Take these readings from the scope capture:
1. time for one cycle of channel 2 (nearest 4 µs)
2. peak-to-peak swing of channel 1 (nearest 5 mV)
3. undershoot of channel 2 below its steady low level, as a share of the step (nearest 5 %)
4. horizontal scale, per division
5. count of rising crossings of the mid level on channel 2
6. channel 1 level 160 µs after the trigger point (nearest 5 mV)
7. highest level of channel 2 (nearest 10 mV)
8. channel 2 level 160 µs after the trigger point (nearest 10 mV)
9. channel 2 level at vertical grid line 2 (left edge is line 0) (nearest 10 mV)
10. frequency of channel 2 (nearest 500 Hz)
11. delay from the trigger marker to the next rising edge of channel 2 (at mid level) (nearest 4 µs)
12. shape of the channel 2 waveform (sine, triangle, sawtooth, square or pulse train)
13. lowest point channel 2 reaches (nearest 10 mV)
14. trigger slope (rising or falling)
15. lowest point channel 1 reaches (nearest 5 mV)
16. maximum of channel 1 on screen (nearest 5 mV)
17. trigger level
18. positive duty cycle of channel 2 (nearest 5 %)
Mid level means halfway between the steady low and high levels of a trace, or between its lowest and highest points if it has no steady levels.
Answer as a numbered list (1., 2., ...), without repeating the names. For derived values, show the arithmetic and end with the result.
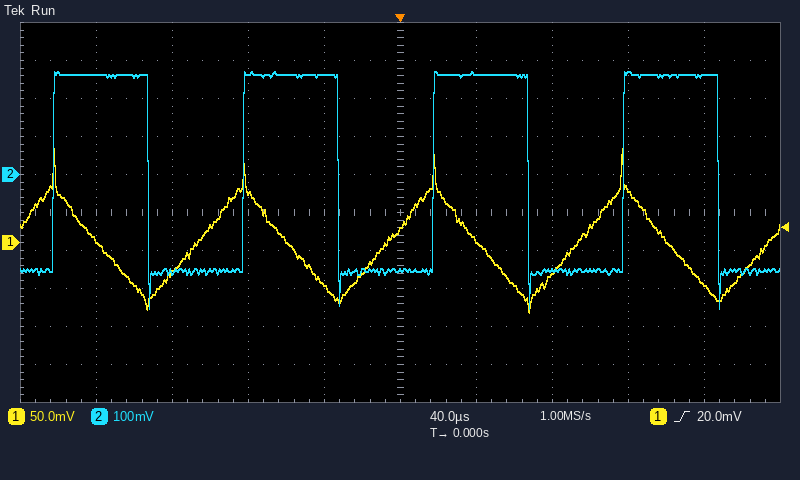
1. 100 µs
2. 125 mV − (-90 mV) = 215 mV
3. 20 %
4. 40 µs
5. 4
6. -55 mV
7. 270 mV
8. 260 mV
9. -260 mV
10. 1 / 100 µs ≈ 10.0 kHz
11. 16 µs
12. square
13. -350 mV
14. rising
15. -90 mV
16. 125 mV
17. 20.0 mV
18. 50 %
